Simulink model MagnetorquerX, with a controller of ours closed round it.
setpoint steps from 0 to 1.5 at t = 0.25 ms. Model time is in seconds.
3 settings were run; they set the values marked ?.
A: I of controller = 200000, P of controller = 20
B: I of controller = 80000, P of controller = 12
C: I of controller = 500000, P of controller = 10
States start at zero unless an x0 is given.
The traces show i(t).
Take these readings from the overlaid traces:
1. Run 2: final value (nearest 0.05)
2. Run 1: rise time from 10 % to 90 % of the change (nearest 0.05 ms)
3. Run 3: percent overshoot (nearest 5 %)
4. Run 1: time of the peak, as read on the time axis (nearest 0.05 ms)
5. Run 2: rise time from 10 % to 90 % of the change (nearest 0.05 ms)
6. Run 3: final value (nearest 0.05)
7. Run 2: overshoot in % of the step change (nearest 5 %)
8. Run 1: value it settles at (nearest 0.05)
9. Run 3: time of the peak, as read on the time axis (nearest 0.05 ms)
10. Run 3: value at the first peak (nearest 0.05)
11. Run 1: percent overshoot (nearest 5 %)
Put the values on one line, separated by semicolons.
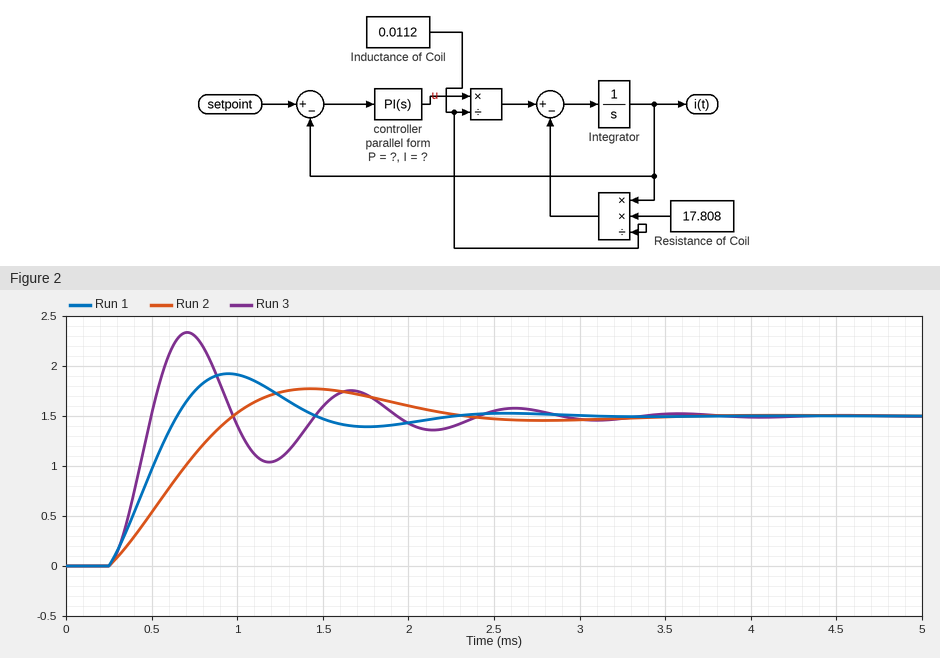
1.50; 0.30 ms; 55 %; 0.95 ms; 0.55 ms; 1.50; 20 %; 1.50; 0.70 ms; 2.35; 30 %
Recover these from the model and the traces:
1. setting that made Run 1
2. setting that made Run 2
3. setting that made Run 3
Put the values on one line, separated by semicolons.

A; B; C
